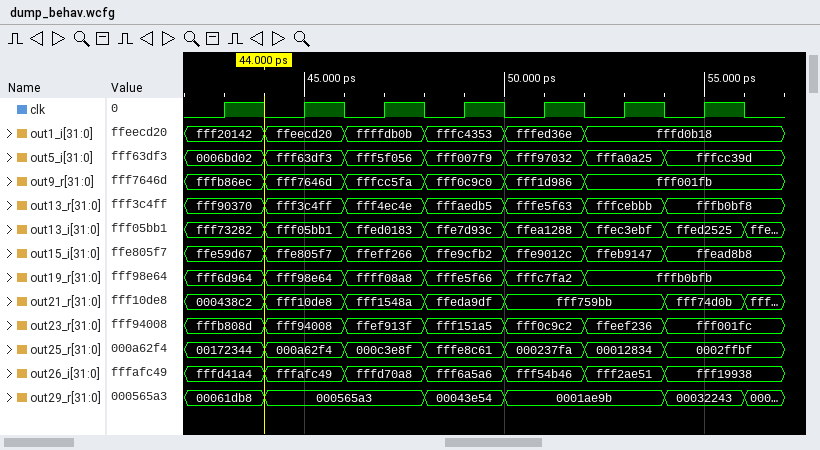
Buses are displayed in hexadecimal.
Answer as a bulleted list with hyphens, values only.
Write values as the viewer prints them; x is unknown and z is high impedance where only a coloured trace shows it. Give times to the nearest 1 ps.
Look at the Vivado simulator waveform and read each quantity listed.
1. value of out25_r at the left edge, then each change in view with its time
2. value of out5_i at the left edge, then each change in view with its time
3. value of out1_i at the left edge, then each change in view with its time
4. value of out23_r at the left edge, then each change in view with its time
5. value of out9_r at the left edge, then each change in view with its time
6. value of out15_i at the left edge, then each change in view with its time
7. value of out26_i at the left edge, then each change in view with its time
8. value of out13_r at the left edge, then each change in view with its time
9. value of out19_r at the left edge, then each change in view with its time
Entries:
- 00172344, 000a62f4 at 44 ps, 000c3e8f at 46 ps, fffe8c61 at 48 ps, 000237fa at 50 ps, 00012834 at 52 ps, 0002ffbf at 54 ps
- 0006bd02, fff63df3 at 44 ps, fff5f056 at 46 ps, fff007f9 at 48 ps, fff97032 at 50 ps, fffa0a25 at 52 ps, fffcc39d at 54 ps
- fff20142, ffeecd20 at 44 ps, ffffdb0b at 46 ps, fffc4353 at 48 ps, fffed36e at 50 ps, fffd0b18 at 52 ps
- fffb808d, fff94008 at 44 ps, ffef913f at 46 ps, fff151a5 at 48 ps, fff0c9c2 at 50 ps, ffeef236 at 52 ps, fff001fc at 54 ps
- fffb86ec, fff7646d at 44 ps, fffcc5fa at 46 ps, fff0c9c0 at 48 ps, fff1d986 at 50 ps, fff001fb at 52 ps
- ffe59d67, ffe805f7 at 44 ps, ffeff266 at 46 ps, ffe9cfb2 at 48 ps, ffe9012c at 50 ps, ffeb9147 at 52 ps, ffead8b8 at 54 ps
- fffd41a4, fffafc49 at 44 ps, fffd70a8 at 46 ps, fff6a5a6 at 48 ps, fff54b46 at 50 ps, fff2ae51 at 52 ps, fff19938 at 54 ps
- fff90370, fff3c4ff at 44 ps, fff4ec4e at 46 ps, fffaedb5 at 48 ps, fffe5f63 at 50 ps, fffcebbb at 52 ps, fffb0bf8 at 54 ps
- fff6d964, fff98e64 at 44 ps, ffff08a8 at 46 ps, fffe5f66 at 48 ps, fffc7fa2 at 50 ps, fffb0bfb at 52 ps
